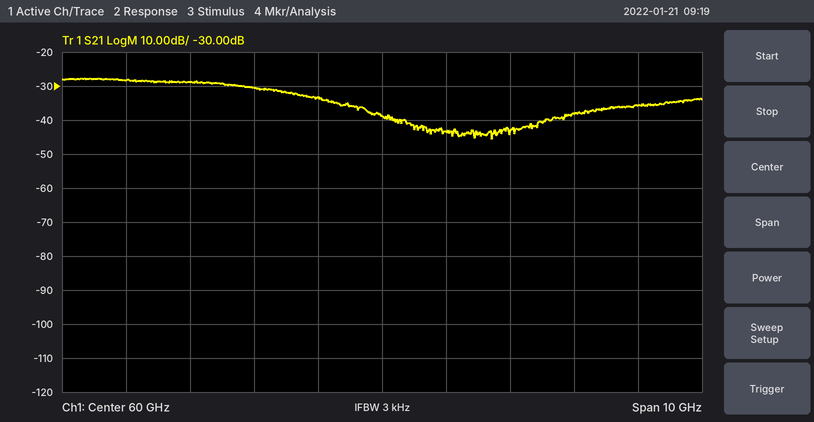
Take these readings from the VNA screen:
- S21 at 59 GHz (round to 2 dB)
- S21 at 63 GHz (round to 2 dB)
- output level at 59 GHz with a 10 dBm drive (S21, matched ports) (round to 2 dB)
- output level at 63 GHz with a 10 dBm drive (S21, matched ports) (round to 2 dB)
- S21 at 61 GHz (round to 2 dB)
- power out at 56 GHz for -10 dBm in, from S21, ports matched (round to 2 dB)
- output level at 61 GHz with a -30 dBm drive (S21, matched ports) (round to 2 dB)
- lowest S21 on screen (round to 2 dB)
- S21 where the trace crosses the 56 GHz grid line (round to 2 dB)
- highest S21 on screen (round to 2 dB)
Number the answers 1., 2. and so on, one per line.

1. -34 dB
2. -38 dB
3. -24 dBm
4. -28 dBm
5. -44 dB
6. -38 dBm
7. -74 dBm
8. -46 dB
9. -28 dB
10. -28 dB
